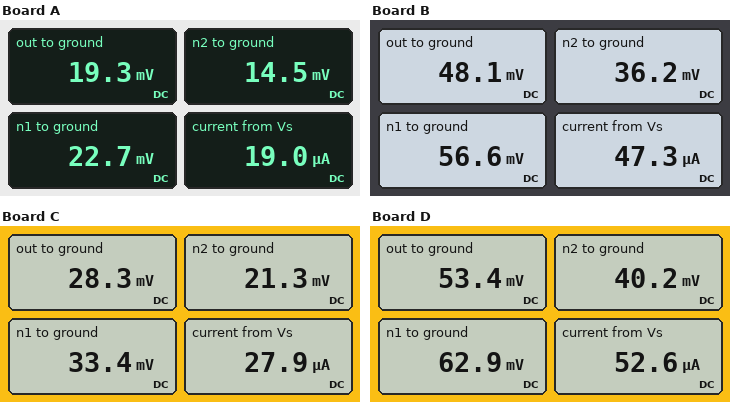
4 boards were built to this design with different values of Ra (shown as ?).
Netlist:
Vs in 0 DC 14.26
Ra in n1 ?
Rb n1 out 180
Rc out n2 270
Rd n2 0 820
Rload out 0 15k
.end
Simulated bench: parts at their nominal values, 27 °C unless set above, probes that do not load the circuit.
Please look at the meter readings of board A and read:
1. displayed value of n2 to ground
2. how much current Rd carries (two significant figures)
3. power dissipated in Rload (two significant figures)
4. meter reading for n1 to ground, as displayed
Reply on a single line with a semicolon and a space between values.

14.5 mV; 18 µA; 25 nW; 22.7 mV
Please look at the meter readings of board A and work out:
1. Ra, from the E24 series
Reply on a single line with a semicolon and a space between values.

750 kΩ
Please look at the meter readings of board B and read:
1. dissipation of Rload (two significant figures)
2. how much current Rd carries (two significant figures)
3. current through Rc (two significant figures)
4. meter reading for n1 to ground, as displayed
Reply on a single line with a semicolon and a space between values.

150 nW; 44 µA; 44 µA; 56.6 mV
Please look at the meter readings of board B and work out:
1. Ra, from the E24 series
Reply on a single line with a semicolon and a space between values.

300 kΩ
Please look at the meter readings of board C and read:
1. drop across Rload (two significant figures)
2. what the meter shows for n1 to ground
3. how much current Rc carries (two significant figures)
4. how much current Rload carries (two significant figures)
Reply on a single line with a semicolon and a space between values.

28 mV; 33.4 mV; 26 µA; 1.9 µA
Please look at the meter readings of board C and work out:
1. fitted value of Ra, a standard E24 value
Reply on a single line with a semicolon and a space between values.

510 kΩ
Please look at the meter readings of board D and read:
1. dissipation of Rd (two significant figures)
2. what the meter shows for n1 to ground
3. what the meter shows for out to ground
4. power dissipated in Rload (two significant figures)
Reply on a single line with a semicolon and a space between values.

2.0 µW; 62.9 mV; 53.4 mV; 190 nW
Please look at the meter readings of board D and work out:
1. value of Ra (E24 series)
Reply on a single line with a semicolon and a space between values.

270 kΩ
